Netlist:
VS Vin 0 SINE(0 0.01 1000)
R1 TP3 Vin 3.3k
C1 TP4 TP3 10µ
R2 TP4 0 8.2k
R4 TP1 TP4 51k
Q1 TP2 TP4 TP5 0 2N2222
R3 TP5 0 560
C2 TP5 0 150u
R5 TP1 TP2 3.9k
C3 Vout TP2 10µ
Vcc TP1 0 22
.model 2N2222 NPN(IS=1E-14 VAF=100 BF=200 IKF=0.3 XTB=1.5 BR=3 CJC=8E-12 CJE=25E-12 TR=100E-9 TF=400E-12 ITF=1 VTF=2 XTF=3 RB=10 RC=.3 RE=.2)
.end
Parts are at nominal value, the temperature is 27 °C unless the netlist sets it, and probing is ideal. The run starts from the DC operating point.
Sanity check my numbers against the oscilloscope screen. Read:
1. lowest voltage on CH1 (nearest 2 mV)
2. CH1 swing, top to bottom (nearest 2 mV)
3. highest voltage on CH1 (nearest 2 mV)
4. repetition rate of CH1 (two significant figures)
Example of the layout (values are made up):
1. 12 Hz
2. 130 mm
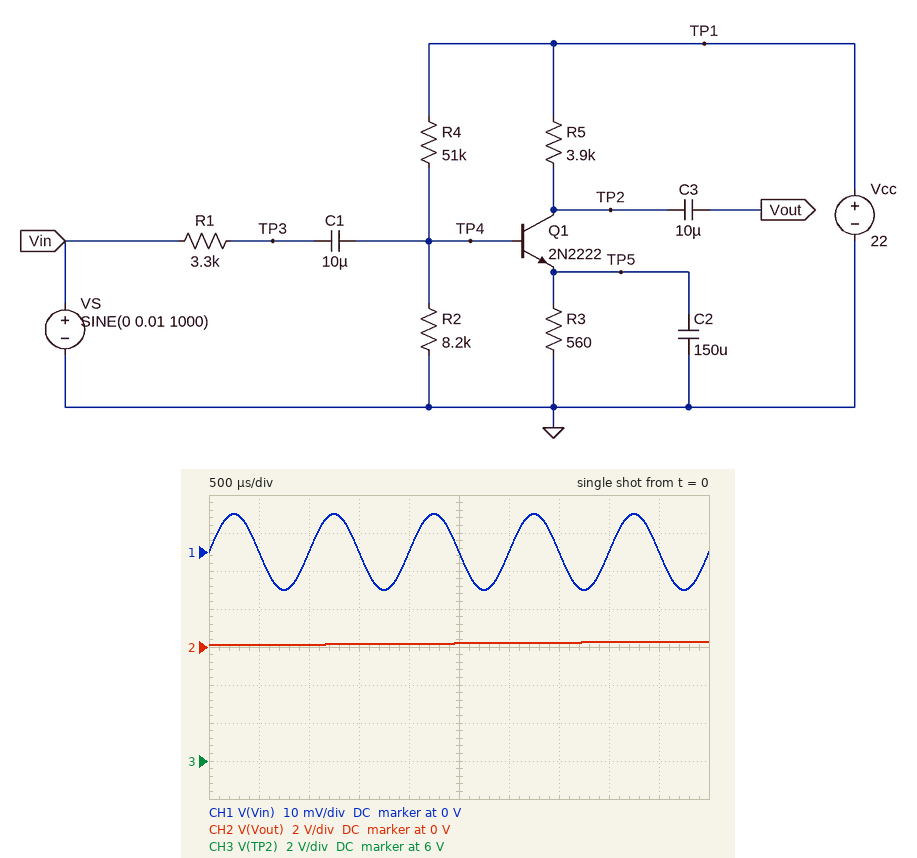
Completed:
1. -10 mV
2. 20 mV
3. 10 mV
4. 1.0 kHz
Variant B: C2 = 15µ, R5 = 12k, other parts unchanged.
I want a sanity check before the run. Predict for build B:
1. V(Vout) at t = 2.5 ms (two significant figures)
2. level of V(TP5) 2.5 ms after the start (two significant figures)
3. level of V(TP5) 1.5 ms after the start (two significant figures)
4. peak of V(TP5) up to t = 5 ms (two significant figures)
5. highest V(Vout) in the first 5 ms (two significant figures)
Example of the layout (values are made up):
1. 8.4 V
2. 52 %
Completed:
1. 360 mV
2. 270 mV
3. 180 mV
4. 390 mV
5. 12 V
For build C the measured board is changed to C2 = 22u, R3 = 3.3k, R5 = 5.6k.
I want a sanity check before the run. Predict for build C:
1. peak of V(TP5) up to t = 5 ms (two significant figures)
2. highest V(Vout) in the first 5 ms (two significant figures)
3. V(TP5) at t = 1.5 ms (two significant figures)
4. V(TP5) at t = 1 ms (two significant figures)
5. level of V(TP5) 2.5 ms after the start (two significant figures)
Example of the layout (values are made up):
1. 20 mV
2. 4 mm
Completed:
1. 420 mV
2. 19 V
3. 270 mV
4. 180 mV
5. 350 mV
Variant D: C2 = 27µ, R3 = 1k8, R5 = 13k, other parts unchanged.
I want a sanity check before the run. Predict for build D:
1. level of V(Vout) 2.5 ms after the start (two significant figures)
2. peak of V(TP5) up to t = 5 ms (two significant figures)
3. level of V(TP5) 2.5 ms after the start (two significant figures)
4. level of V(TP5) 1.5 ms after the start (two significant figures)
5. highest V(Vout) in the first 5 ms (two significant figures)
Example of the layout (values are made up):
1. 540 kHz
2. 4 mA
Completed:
1. 220 mV
2. 310 mV
3. 160 mV
4. 99 mV
5. 390 mV
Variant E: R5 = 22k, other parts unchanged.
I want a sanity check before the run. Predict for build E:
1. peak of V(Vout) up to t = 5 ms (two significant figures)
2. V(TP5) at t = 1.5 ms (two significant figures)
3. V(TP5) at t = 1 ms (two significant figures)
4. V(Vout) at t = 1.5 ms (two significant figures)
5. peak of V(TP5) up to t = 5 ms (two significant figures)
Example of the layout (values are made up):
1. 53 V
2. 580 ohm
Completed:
1. 72 mV
2. 11 mV
3. 7.6 mV
4. 47 mV
5. 37 mV
